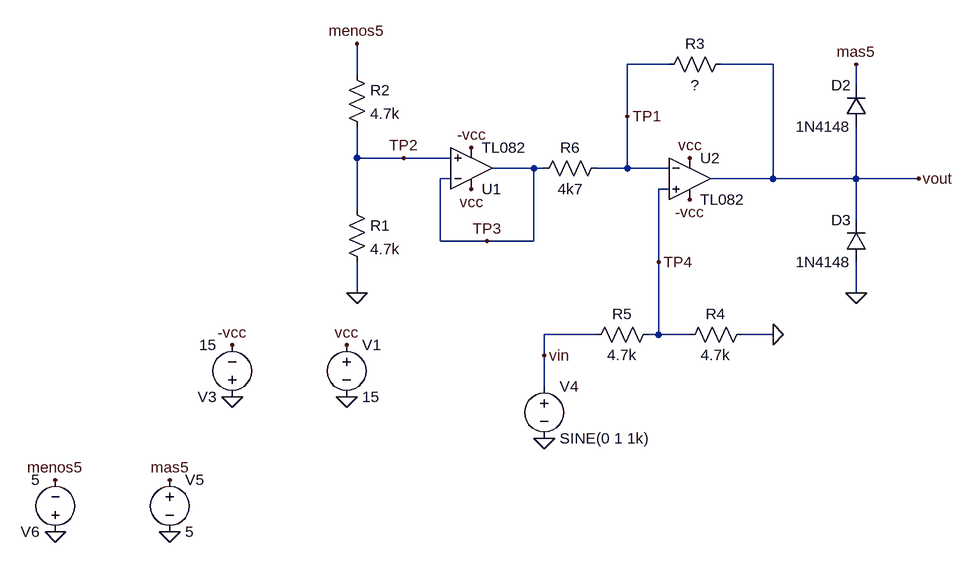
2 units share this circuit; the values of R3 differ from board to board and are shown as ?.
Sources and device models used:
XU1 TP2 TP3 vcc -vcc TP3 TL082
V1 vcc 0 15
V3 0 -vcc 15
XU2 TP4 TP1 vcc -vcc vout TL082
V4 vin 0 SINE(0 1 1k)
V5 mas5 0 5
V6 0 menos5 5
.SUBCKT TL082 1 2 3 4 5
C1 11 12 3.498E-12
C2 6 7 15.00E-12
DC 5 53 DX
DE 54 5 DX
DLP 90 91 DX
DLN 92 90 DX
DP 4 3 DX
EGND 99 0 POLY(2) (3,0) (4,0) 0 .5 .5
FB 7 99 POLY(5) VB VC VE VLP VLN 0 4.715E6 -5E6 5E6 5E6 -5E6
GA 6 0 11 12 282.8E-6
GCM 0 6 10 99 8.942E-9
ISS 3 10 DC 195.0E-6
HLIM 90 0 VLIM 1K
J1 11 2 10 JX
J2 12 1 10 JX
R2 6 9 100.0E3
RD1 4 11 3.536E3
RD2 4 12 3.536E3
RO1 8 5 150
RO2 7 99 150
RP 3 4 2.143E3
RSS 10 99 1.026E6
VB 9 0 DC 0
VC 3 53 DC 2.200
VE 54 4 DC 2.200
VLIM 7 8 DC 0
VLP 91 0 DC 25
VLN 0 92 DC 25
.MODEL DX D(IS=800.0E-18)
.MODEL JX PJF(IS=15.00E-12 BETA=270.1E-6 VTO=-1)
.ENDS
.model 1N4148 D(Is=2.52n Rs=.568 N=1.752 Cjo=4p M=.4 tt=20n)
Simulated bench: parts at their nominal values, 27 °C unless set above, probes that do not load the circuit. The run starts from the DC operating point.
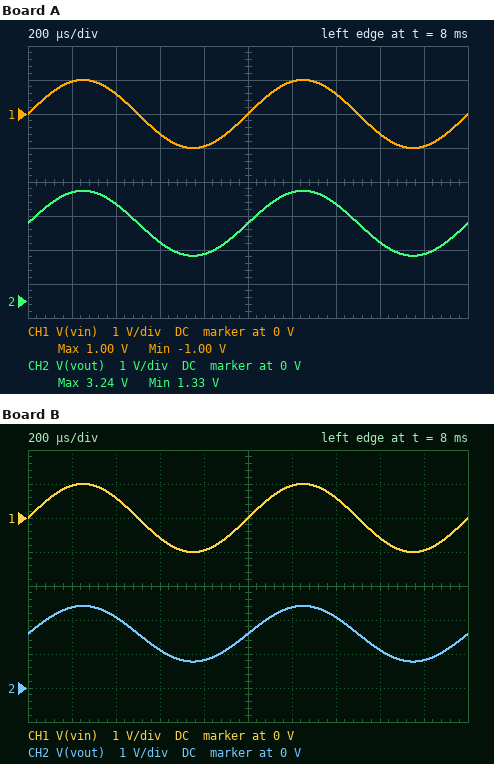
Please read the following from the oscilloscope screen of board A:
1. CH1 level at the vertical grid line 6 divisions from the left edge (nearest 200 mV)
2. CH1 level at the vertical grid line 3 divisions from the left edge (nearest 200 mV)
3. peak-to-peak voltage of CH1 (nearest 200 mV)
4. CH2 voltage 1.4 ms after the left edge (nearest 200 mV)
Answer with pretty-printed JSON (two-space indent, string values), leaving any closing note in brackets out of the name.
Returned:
{
  "CH1 level at the vertical grid line 6 divisions from the left edge": "1.0 V",
  "CH1 level at the vertical grid line 3 divisions from the left edge": "-600 mV",
  "peak-to-peak voltage of CH1": "2.0 V",
  "CH2 voltage 1.4 ms after the left edge": "2.8 V"
}
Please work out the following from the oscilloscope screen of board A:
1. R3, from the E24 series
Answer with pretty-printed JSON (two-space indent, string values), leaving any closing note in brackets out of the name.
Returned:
{
  "R3, from the E24 series": "4.3 kΩ"
}
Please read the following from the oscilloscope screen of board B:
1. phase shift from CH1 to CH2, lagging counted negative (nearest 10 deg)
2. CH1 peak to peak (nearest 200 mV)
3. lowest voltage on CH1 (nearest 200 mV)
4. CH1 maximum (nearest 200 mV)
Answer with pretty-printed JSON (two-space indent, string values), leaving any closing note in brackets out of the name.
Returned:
{
  "phase shift from CH1 to CH2, lagging counted negative": "0 deg",
  "CH1 peak to peak": "2.0 V",
  "lowest voltage on CH1": "-1.0 V",
  "CH1 maximum": "1.0 V"
}
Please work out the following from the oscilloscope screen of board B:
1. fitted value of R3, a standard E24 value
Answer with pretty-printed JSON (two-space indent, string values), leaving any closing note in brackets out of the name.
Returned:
{
  "fitted value of R3, a standard E24 value": "3 kΩ"
}
